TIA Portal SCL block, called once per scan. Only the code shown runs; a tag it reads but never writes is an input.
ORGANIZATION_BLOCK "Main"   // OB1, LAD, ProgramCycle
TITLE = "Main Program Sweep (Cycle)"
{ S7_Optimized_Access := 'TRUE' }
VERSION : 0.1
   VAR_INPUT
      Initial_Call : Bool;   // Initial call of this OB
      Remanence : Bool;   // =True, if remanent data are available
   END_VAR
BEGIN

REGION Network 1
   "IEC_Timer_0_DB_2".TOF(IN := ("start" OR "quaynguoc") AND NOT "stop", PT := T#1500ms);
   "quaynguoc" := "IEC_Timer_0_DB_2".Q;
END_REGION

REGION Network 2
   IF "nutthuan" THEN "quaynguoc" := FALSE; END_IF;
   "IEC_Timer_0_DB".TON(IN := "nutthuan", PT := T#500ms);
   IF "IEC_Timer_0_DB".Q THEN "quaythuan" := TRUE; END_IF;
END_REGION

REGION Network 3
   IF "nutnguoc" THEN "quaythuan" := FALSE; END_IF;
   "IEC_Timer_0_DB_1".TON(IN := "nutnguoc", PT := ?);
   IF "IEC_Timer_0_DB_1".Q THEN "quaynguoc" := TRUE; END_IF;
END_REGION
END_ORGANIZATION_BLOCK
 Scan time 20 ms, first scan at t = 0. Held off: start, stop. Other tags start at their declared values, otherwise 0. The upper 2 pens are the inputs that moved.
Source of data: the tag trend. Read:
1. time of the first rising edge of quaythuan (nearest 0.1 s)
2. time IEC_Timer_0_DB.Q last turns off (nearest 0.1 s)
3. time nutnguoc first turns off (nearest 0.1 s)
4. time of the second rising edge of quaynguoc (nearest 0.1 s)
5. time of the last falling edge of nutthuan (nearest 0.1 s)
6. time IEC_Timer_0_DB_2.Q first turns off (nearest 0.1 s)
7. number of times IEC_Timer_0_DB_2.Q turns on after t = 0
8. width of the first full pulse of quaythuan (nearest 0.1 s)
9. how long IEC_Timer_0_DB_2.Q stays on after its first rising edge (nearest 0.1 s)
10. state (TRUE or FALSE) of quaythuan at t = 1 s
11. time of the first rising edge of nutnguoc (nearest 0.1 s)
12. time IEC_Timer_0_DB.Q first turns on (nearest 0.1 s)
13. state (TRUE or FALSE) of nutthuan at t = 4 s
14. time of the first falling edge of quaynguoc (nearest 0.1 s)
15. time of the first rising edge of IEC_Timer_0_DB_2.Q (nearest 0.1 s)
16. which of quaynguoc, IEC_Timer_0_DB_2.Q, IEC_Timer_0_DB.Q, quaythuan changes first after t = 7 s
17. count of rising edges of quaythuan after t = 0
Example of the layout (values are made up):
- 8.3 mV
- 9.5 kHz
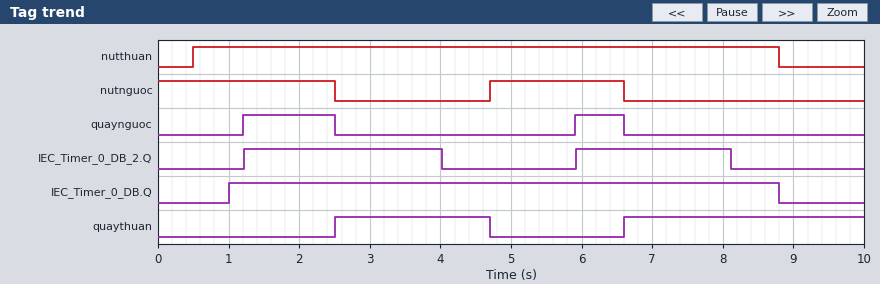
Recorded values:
- 2.5 s
- 8.8 s
- 2.5 s
- 5.9 s
- 8.8 s
- 4.0 s
- 2
- 2.2 s
- 2.8 s
- FALSE
- 4.7 s
- 1.0 s
- TRUE
- 2.5 s
- 1.2 s
- IEC_Timer_0_DB_2.Q
- 2
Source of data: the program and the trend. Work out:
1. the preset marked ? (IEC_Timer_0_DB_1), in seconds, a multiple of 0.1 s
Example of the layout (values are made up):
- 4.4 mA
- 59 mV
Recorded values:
- 1.2 s
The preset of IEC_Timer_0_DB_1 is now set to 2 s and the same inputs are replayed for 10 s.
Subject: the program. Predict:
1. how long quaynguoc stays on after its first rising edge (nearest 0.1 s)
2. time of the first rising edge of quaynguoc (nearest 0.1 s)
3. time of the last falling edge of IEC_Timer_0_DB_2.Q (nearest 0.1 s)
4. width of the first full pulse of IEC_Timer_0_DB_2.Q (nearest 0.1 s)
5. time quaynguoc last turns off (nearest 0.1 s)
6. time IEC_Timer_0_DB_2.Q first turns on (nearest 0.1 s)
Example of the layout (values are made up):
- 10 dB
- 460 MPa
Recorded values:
- 0.5 s
- 2.0 s
- 4.0 s
- 2.0 s
- 2.5 s
- 2.0 s
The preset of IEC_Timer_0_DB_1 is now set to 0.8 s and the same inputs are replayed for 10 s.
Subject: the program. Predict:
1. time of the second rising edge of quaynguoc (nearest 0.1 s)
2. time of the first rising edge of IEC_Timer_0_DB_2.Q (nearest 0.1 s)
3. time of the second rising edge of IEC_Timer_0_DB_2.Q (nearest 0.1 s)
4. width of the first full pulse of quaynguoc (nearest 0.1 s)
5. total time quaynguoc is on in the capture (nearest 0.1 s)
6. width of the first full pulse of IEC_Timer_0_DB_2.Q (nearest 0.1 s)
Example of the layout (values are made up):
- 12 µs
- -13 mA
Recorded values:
- 5.5 s
- 0.8 s
- 5.5 s
- 1.7 s
- 2.8 s
- 3.2 s
